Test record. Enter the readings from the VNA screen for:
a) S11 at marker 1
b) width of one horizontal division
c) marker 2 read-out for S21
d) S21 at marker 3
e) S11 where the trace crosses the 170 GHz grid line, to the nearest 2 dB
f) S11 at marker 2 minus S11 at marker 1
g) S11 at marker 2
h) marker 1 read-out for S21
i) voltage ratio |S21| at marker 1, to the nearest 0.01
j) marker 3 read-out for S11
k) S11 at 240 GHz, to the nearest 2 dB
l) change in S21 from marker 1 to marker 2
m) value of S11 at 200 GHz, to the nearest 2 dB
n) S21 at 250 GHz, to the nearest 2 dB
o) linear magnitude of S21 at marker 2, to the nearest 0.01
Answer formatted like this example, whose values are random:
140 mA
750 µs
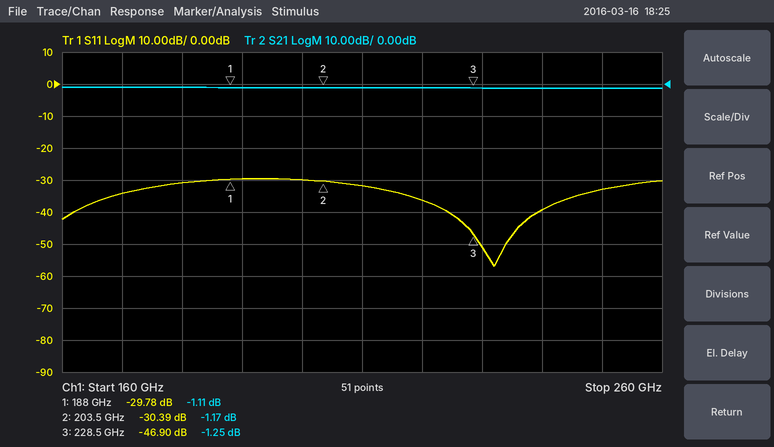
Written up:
-29.78 dB
10 GHz
-1.17 dB
-1.25 dB
-34 dB
-0.61 dB
-30.39 dB
-1.11 dB
0.88
-46.90 dB
-40 dB
-0.06 dB
-30 dB
-2 dB
0.87
